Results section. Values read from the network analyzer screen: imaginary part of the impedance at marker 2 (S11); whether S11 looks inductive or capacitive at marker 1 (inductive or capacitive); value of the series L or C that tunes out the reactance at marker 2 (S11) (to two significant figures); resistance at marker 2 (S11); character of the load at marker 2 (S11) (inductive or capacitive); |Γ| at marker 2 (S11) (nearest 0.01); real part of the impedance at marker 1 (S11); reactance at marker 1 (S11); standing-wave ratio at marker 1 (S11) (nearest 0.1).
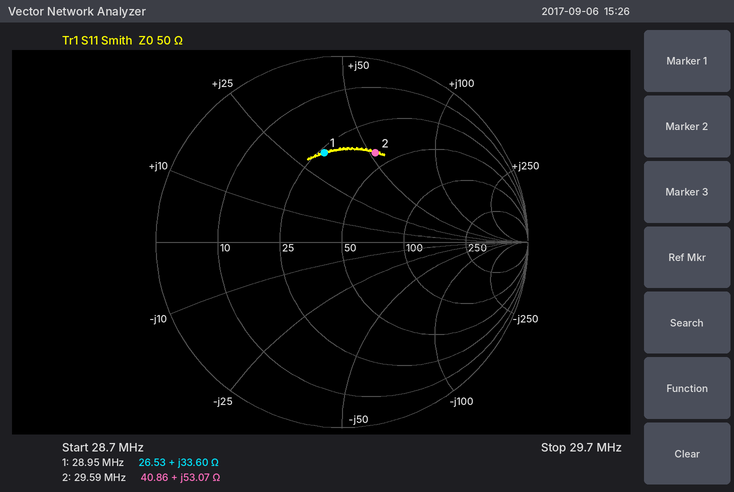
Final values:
+53.07 Ω
inductive
100 pF
40.86 Ω
inductive
0.51
26.53 Ω
+33.60 Ω
2.9
